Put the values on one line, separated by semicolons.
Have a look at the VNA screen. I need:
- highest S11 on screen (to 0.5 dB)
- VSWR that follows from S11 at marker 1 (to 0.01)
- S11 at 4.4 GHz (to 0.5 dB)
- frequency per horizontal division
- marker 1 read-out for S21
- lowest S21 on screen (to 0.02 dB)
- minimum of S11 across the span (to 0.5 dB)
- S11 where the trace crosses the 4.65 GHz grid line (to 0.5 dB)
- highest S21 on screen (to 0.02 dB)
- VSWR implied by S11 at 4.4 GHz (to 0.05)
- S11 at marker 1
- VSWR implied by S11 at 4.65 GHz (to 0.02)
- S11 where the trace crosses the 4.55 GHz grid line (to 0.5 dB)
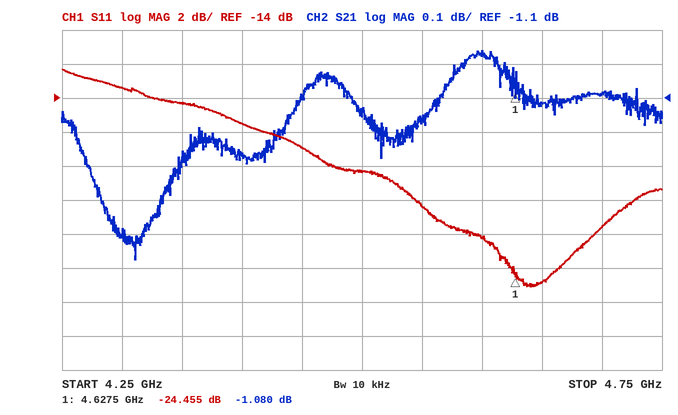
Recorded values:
-12.5 dB; 1.13; -15.5 dB; 50 MHz; -1.080 dB; -1.58 dB; -25.0 dB; -25.0 dB; -0.96 dB; 1.40; -24.455 dB; 1.12; -20.5 dB
